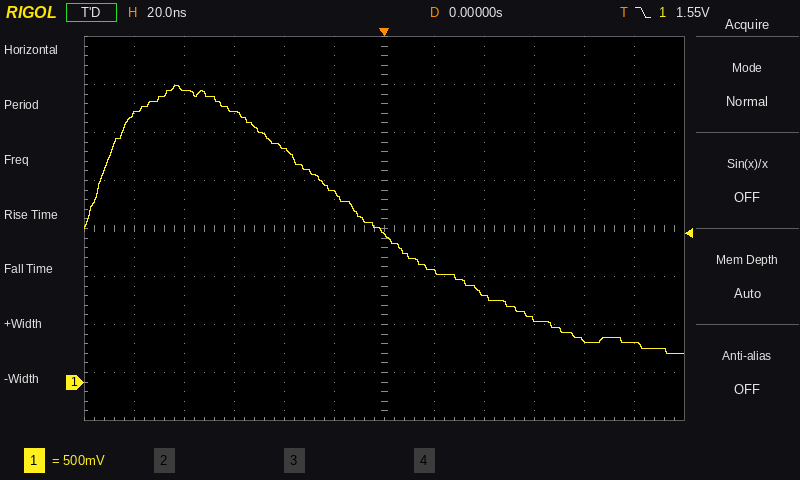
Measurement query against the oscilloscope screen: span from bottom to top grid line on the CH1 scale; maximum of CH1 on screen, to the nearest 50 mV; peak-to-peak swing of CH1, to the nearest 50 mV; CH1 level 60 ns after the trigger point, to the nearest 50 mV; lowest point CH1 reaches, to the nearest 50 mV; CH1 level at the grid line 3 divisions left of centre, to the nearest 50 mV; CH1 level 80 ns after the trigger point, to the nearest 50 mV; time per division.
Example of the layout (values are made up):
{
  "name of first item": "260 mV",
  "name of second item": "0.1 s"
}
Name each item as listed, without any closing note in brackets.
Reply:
{
  "span from bottom to top grid line on the CH1 scale": "4 V",
  "maximum of CH1 on screen, to the nearest 50 mV": "3.10 V",
  "peak-to-peak swing of CH1, to the nearest 50 mV": "2.80 V",
  "CH1 level 60 ns after the trigger point, to the nearest 50 mV": "650 mV",
  "lowest point CH1 reaches, to the nearest 50 mV": "300 mV",
  "CH1 level at the grid line 3 divisions left of centre, to the nearest 50 mV": "2.80 V",
  "CH1 level 80 ns after the trigger point, to the nearest 50 mV": "450 mV",
  "time per division": "20 ns"
}
